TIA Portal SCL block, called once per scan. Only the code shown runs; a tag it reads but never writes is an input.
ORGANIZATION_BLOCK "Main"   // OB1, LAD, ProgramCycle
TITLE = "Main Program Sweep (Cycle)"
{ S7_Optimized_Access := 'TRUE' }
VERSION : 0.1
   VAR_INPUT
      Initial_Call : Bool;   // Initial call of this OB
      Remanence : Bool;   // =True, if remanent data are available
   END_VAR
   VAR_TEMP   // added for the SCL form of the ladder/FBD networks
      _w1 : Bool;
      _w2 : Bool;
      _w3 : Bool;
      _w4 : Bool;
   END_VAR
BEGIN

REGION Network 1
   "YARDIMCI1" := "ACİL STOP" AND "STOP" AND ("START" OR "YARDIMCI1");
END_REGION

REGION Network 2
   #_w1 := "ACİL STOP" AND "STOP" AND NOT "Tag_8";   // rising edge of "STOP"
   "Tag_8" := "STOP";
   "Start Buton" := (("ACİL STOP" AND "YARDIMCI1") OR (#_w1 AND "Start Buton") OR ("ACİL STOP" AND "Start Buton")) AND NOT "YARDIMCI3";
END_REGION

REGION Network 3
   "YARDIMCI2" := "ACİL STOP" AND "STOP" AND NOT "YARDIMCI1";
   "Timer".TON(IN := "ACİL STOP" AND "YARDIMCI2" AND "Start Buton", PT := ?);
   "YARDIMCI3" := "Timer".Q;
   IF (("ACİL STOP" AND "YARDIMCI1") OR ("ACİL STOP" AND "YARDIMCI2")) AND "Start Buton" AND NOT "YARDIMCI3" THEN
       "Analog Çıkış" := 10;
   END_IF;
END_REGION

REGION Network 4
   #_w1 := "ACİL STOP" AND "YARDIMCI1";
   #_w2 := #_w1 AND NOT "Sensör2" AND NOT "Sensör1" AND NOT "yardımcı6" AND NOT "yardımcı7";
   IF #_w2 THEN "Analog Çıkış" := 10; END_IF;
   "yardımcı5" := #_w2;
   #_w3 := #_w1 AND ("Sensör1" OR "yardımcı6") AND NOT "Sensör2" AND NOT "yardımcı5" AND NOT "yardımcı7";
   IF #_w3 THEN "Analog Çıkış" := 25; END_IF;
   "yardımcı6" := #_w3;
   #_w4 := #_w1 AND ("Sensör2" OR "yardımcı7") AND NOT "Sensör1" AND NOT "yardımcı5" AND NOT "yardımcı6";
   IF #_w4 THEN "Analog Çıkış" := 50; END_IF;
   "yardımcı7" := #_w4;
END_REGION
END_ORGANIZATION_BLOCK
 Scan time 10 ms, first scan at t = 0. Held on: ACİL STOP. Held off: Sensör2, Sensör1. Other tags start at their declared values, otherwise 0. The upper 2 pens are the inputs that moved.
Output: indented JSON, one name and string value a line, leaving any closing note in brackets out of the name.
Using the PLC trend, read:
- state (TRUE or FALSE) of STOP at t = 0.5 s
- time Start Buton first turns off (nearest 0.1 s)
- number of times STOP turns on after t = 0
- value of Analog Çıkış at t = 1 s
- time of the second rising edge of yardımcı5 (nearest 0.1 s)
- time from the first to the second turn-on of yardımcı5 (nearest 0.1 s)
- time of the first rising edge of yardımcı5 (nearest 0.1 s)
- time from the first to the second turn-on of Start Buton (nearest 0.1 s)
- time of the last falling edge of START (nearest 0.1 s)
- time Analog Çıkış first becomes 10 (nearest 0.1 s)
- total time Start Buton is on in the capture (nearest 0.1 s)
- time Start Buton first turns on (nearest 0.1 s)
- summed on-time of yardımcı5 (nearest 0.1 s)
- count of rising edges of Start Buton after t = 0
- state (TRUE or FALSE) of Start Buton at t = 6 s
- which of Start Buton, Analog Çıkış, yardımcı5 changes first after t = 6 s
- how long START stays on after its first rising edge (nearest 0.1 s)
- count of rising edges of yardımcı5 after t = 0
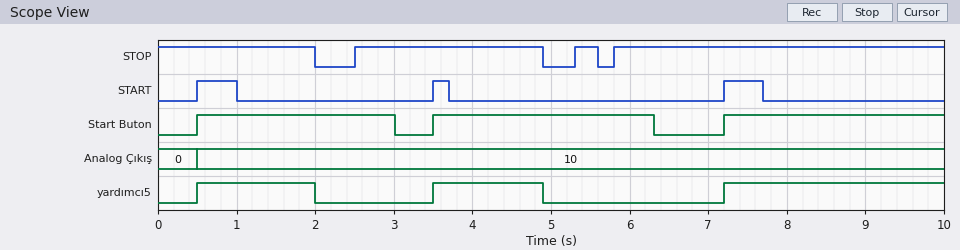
{
  "state (TRUE or FALSE) of STOP at t = 0.5 s": "TRUE",
  "time Start Buton first turns off": "3.0 s",
  "number of times STOP turns on after t = 0": "3",
  "value of Analog Çıkış at t = 1 s": "10",
  "time of the second rising edge of yardımcı5": "3.5 s",
  "time from the first to the second turn-on of yardımcı5": "3.0 s",
  "time of the first rising edge of yardımcı5": "0.5 s",
  "time from the first to the second turn-on of Start Buton": "3.0 s",
  "time of the last falling edge of START": "7.7 s",
  "time Analog Çıkış first becomes 10": "0.5 s",
  "total time Start Buton is on in the capture": "8.1 s",
  "time Start Buton first turns on": "0.5 s",
  "summed on-time of yardımcı5": "5.7 s",
  "count of rising edges of Start Buton after t = 0": "3",
  "state (TRUE or FALSE) of Start Buton at t = 6 s": "TRUE",
  "which of Start Buton, Analog Çıkış, yardımcı5 changes first after t = 6 s": "Start Buton",
  "how long START stays on after its first rising edge": "0.5 s",
  "count of rising edges of yardımcı5 after t = 0": "3"
}
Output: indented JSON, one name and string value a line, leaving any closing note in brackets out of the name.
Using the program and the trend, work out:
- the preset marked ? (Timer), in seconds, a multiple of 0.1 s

{
  "the preset marked ? (Timer), in seconds, a multiple of 0.1 s": "0.5 s"
}
